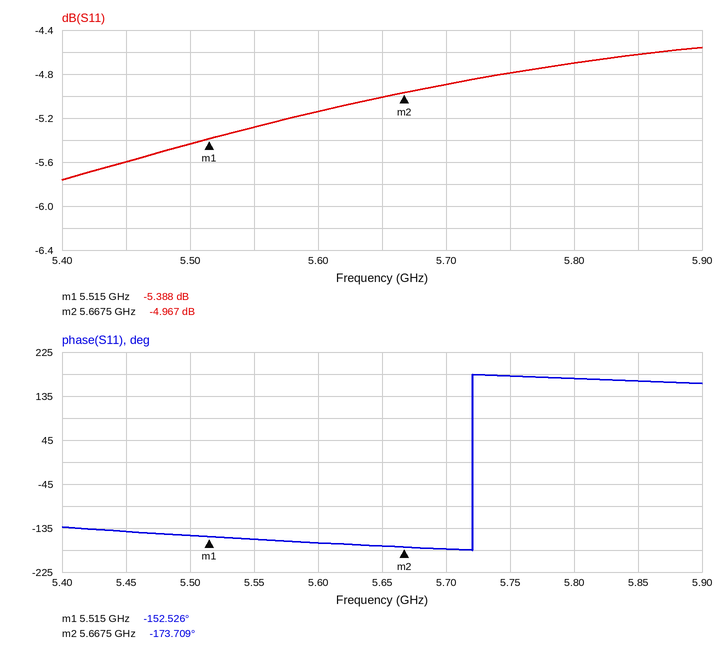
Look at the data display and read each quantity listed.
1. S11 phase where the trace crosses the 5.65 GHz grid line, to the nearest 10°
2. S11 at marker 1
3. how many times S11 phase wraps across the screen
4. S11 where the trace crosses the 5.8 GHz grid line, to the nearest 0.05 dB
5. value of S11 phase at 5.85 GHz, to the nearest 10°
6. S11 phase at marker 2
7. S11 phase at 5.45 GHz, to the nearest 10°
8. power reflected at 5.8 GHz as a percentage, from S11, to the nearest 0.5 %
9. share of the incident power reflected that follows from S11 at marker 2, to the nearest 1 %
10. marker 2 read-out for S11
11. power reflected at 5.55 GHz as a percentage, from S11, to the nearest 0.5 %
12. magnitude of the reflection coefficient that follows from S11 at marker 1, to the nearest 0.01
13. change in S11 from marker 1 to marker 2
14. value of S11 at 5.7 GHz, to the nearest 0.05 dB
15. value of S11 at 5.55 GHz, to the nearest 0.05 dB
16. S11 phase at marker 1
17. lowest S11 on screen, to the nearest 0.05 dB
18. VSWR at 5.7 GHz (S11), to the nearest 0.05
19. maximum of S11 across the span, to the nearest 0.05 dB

-170°
-5.388 dB
1
-4.70 dB
170°
-173.709°
-140°
34.0 %
32 %
-4.967 dB
29.5 %
0.54
0.421 dB
-4.90 dB
-5.30 dB
-152.526°
-5.75 dB
3.65
-4.55 dB
